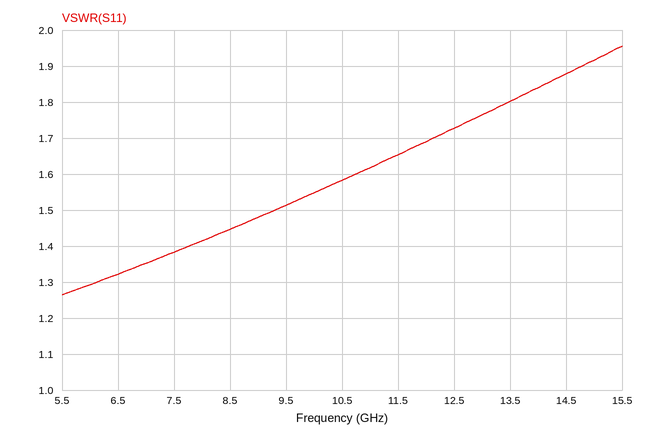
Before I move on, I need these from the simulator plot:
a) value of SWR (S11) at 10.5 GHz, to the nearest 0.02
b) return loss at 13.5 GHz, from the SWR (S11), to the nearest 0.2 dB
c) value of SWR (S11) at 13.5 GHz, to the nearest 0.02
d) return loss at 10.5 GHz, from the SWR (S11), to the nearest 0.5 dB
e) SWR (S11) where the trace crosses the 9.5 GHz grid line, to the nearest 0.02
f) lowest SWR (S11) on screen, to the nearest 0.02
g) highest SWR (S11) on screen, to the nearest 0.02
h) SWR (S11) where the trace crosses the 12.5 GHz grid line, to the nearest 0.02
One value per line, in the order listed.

1.58
10.8 dB
1.80
13.0 dB
1.52
1.26
1.96
1.72
